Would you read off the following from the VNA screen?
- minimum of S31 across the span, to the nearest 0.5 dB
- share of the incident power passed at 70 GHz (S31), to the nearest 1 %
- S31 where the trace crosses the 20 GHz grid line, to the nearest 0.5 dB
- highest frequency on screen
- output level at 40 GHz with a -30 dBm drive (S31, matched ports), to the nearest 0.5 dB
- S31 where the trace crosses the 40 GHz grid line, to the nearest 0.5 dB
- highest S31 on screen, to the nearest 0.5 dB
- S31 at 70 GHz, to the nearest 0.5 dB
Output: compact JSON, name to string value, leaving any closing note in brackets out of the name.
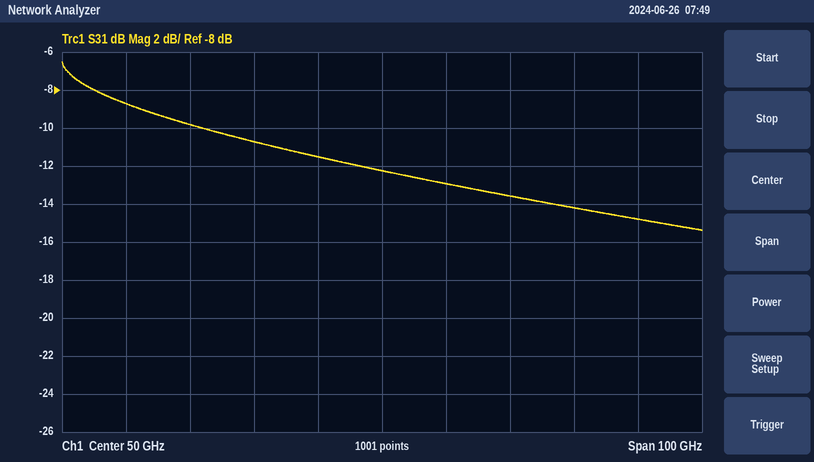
{"minimum of S31 across the span, to the nearest 0.5 dB": "-15.5 dB", "share of the incident power passed at 70 GHz (S31), to the nearest 1 %": "4 %", "S31 where the trace crosses the 20 GHz grid line, to the nearest 0.5 dB": "-10.0 dB", "highest frequency on screen": "100 GHz", "output level at 40 GHz with a -30 dBm drive (S31, matched ports), to the nearest 0.5 dB": "-41.5 dBm", "S31 where the trace crosses the 40 GHz grid line, to the nearest 0.5 dB": "-11.5 dB", "highest S31 on screen, to the nearest 0.5 dB": "-6.5 dB", "S31 at 70 GHz, to the nearest 0.5 dB": "-13.5 dB"}
